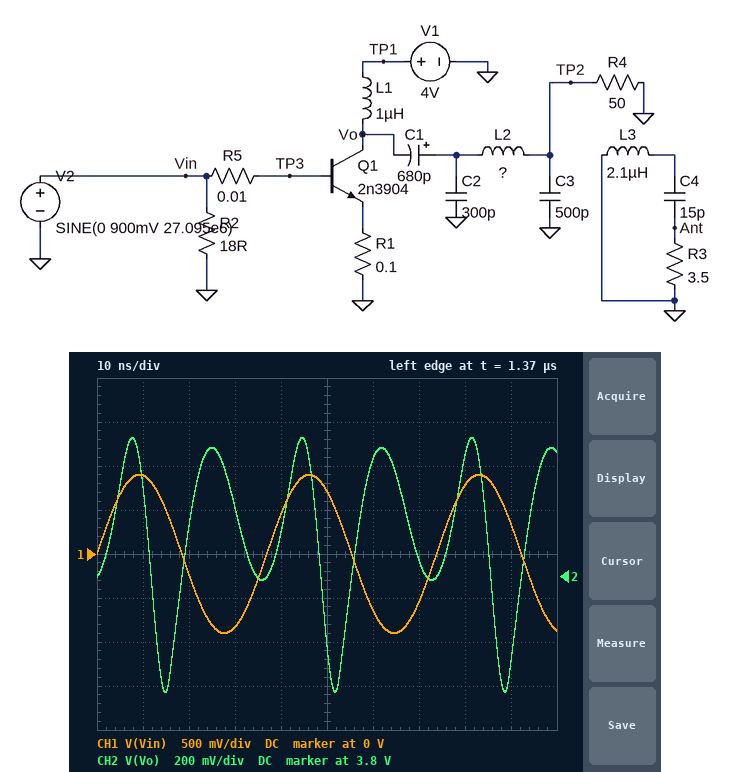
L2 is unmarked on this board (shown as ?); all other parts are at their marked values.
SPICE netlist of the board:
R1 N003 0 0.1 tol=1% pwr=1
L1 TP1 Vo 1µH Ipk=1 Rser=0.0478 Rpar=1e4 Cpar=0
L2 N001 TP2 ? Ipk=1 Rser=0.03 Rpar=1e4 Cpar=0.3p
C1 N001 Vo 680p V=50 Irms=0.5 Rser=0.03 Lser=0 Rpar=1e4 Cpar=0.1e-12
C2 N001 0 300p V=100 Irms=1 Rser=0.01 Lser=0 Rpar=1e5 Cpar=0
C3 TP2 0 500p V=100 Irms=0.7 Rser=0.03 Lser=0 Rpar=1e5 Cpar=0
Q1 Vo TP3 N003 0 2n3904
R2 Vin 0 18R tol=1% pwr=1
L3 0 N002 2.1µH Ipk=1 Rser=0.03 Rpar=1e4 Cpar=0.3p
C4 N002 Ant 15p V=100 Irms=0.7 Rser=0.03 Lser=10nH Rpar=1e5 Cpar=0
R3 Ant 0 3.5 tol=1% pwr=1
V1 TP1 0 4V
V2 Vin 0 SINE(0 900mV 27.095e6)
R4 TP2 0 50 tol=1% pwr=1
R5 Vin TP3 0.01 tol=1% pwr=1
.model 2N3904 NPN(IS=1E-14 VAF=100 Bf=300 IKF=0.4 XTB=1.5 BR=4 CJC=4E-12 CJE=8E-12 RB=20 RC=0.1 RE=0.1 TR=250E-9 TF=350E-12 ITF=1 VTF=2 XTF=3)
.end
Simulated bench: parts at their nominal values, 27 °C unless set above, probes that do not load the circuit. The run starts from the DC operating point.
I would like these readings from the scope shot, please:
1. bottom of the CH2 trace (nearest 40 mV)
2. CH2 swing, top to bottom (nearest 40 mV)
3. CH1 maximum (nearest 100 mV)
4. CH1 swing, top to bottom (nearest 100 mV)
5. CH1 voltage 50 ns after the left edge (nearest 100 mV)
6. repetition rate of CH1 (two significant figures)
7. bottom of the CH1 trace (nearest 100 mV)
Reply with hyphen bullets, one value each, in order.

- 3.28 V
- 1.16 V
- 900 mV
- 1.8 V
- 700 mV
- 27 MHz
- -900 mV
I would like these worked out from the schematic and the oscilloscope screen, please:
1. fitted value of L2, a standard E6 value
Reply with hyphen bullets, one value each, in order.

- 100 nH
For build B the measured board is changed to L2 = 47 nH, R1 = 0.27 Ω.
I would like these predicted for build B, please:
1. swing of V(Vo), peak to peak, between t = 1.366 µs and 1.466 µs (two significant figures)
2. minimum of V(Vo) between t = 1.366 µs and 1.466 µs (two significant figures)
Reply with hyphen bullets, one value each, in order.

- 4.2 V
- 1.8 V
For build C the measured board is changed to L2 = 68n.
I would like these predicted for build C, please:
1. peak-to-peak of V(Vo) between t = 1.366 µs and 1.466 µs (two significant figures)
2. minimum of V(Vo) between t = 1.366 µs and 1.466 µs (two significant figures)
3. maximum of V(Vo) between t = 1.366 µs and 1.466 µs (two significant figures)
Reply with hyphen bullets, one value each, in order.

- 1.7 V
- 3.1 V
- 4.7 V
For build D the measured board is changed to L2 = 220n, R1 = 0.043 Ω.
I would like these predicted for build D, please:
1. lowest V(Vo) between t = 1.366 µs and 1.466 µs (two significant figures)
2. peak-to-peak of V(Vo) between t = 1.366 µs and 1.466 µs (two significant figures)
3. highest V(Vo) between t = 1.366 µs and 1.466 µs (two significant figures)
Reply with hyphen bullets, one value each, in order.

- 1.1 V
- 5.5 V
- 6.5 V
